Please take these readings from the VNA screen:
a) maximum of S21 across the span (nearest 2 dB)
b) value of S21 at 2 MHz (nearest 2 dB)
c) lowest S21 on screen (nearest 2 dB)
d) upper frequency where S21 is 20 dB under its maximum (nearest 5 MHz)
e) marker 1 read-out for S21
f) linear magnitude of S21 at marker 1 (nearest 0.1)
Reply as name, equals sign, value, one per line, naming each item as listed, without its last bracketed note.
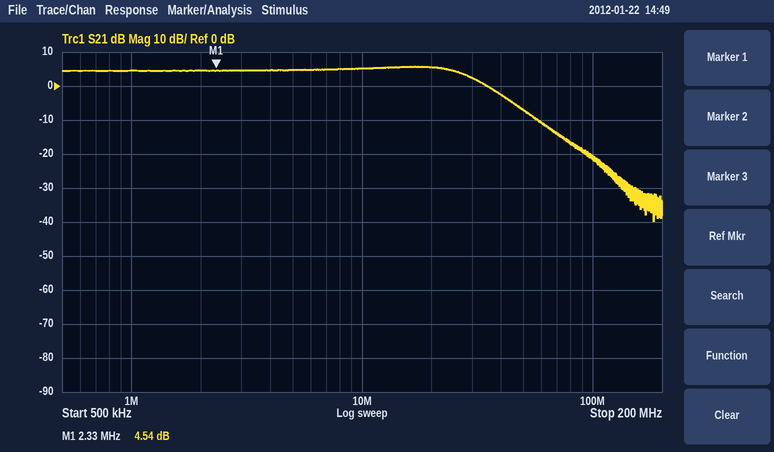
maximum of S21 across the span = 6 dB
value of S21 at 2 MHz = 4 dB
lowest S21 on screen = -40 dB
upper frequency where S21 is 20 dB under its maximum = 70 MHz
marker 1 read-out for S21 = 4.54 dB
linear magnitude of S21 at marker 1 = 1.7
